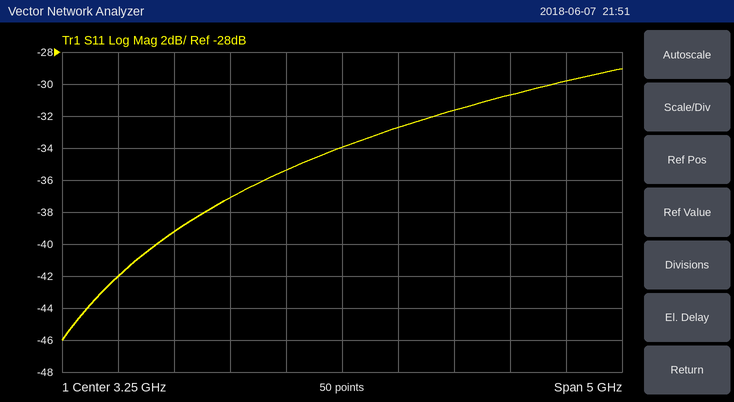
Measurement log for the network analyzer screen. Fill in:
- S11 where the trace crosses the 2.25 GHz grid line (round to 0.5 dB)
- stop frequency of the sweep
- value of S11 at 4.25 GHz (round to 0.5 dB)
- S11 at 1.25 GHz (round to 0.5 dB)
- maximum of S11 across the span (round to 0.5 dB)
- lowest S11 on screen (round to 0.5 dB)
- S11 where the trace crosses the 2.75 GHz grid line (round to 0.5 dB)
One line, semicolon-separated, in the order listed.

-37.0 dB; 5.75 GHz; -31.5 dB; -42.0 dB; -29.0 dB; -46.0 dB; -35.5 dB
